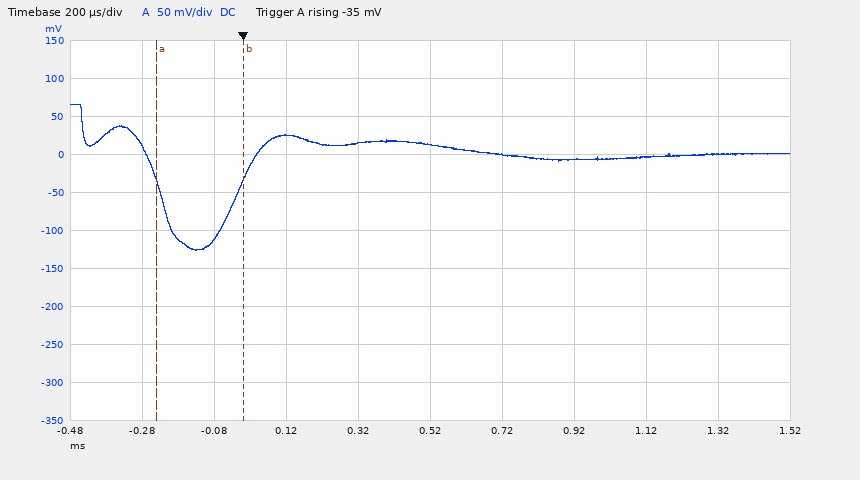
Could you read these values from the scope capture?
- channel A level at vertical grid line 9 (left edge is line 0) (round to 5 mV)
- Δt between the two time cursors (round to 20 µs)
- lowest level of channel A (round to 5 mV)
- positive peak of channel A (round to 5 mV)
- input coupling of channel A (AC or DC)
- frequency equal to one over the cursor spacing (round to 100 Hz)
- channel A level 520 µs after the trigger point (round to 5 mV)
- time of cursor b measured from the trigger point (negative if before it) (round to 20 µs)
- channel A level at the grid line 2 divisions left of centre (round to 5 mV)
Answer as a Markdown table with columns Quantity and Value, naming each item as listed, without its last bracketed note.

| Quantity | Value |
|---|---|
| channel A level at vertical grid line 9 (left edge is line 0) | 0 mV |
| Δt between the two time cursors | 240 µs |
| lowest level of channel A | -125 mV |
| positive peak of channel A | 65 mV |
| input coupling of channel A | DC |
| frequency equal to one over the cursor spacing | 4.2 kHz |
| channel A level 520 µs after the trigger point | 15 mV |
| time of cursor b measured from the trigger point (negative if before it) | 0 µs |
| channel A level at the grid line 2 divisions left of centre | 25 mV |
